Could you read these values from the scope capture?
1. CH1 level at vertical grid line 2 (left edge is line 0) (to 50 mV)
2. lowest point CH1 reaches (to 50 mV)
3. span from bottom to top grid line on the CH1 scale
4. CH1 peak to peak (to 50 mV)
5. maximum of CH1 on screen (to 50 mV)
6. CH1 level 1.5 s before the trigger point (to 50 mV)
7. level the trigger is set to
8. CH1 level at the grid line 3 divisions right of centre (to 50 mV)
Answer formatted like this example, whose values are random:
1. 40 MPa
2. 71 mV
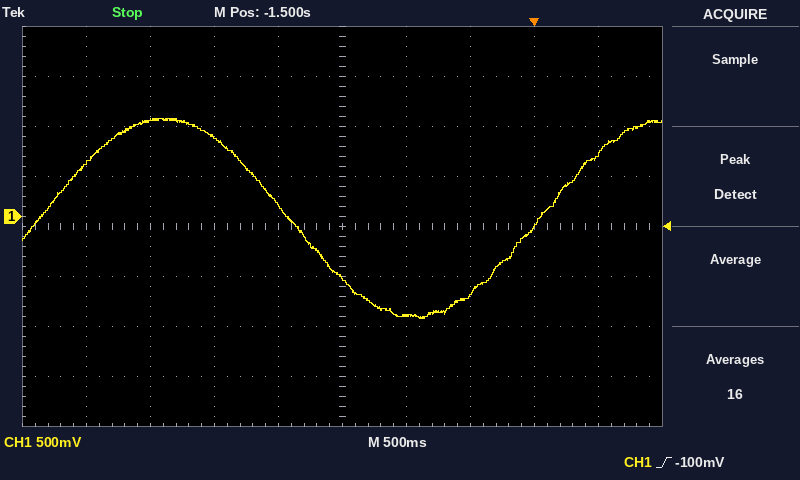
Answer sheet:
1. 950 mV
2. -1.00 V
3. 4 V
4. 2.00 V
5. 1.00 V
6. -600 mV
7. -100 mV
8. -100 mV
